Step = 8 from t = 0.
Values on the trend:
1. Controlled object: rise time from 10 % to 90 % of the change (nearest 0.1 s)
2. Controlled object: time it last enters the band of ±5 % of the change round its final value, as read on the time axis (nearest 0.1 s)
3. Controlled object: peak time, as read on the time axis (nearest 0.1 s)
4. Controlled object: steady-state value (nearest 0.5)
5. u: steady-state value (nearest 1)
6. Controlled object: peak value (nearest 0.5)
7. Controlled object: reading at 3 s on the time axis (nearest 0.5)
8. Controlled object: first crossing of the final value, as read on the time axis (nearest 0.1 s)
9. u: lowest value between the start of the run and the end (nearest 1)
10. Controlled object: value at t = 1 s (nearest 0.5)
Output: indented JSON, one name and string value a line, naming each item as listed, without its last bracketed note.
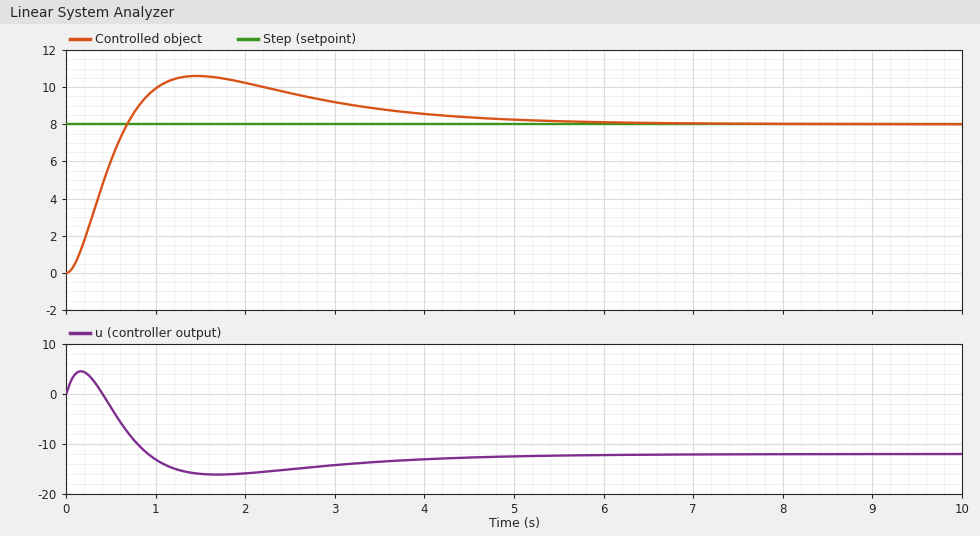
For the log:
{
  "Controlled object: rise time from 10 % to 90 % of the change": "0.5 s",
  "Controlled object: time it last enters the band of ±5 % of the change round its final value, as read on the time axis": "4.4 s",
  "Controlled object: peak time, as read on the time axis": "1.5 s",
  "Controlled object: steady-state value": "8.0",
  "u: steady-state value": "-12",
  "Controlled object: peak value": "10.5",
  "Controlled object: reading at 3 s on the time axis": "9.0",
  "Controlled object: first crossing of the final value, as read on the time axis": "0.7 s",
  "u: lowest value between the start of the run and the end": "-16",
  "Controlled object: value at t = 1 s": "10.0"
}
